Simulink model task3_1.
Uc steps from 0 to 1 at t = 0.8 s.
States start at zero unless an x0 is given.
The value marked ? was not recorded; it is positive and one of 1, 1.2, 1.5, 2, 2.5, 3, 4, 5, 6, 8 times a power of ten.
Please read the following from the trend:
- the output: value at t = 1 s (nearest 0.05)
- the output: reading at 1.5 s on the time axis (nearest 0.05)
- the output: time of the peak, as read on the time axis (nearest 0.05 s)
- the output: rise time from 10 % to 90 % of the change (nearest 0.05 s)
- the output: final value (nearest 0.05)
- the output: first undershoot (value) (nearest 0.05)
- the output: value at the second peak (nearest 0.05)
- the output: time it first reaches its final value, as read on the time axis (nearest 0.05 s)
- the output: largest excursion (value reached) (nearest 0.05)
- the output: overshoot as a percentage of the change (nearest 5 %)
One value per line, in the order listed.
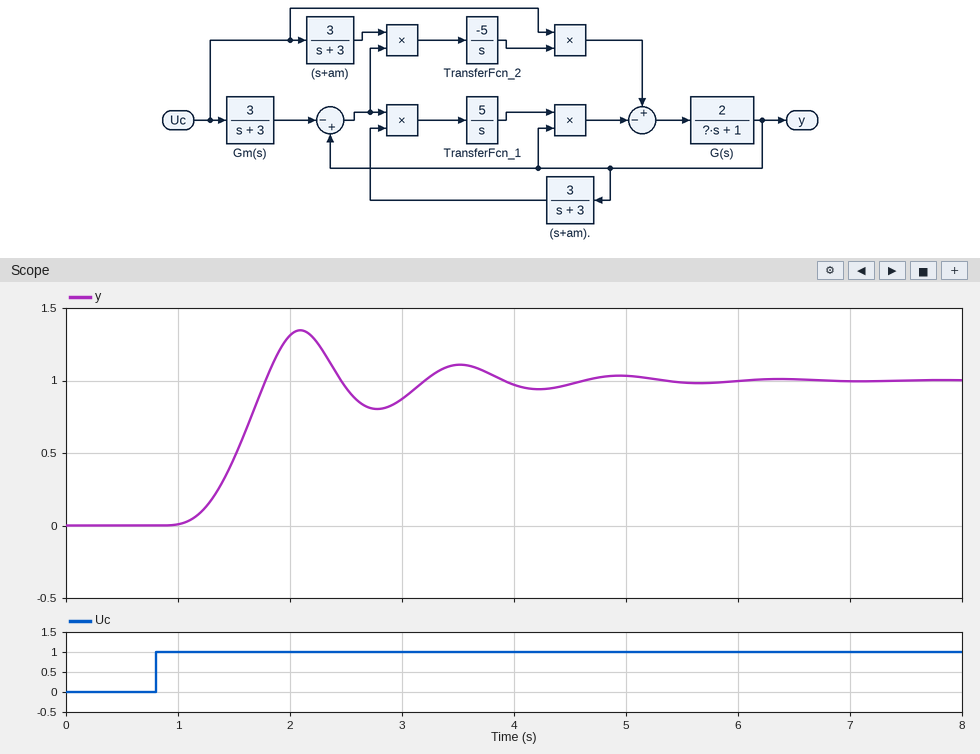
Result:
0.00
0.45
2.10 s
0.50 s
1.00
0.80
1.10
1.80 s
1.35
35 %
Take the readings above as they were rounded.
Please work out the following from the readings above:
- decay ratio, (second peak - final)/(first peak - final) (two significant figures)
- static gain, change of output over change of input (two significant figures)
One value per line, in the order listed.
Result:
0.29
1.0
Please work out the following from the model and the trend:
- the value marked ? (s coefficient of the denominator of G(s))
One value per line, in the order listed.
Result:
1
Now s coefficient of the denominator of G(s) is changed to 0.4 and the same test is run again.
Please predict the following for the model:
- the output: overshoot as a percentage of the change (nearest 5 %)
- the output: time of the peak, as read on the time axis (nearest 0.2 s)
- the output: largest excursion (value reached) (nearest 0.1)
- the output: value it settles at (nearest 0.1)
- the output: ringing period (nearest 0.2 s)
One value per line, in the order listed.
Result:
15 %
1.8 s
1.2
1.0
1.0 s
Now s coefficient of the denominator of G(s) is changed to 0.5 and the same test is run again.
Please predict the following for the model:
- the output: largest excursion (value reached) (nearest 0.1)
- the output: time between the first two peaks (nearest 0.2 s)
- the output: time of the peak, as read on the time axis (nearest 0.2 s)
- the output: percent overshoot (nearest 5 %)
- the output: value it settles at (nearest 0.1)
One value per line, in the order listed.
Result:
1.2
1.0 s
1.8 s
20 %
1.0
